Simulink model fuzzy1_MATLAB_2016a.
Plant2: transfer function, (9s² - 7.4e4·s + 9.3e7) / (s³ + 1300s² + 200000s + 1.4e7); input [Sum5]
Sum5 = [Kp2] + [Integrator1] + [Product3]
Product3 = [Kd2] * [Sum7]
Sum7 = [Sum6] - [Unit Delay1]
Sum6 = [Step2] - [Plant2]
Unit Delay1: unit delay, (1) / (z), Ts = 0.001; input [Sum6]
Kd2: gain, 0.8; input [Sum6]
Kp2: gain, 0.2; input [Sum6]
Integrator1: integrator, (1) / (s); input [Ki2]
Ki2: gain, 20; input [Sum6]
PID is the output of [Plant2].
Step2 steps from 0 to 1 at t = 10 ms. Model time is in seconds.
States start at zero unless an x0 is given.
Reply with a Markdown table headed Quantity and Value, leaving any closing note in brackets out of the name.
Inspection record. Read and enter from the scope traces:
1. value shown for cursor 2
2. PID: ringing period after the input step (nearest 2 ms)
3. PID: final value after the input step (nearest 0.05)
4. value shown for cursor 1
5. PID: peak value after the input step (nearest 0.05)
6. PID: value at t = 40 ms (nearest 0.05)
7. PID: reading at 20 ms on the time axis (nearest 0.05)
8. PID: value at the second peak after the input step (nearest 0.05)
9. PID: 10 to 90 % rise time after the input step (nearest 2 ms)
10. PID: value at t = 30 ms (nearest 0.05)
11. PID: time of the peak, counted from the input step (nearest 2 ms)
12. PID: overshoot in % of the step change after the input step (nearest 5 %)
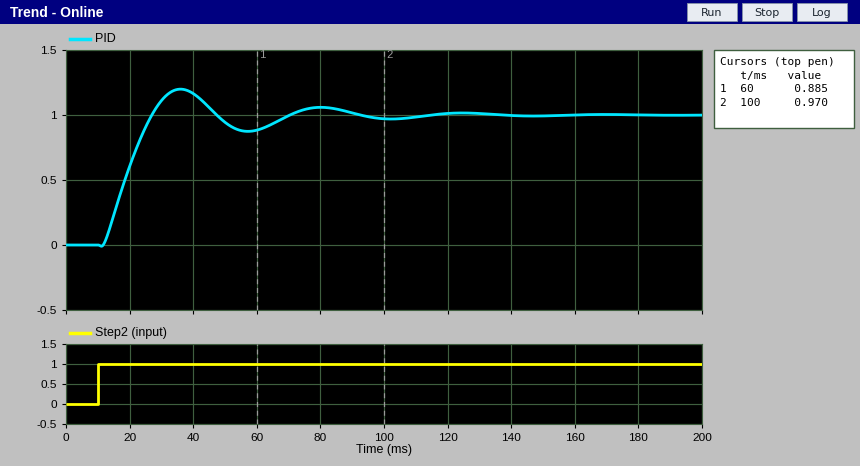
| Quantity | Value |
|---|---|
| value shown for cursor 2 | 0.970 |
| PID: ringing period after the input step | 44 ms |
| PID: final value after the input step | 1.00 |
| value shown for cursor 1 | 0.885 |
| PID: peak value after the input step | 1.20 |
| PID: value at t = 40 ms | 1.15 |
| PID: reading at 20 ms on the time axis | 0.60 |
| PID: value at the second peak after the input step | 1.05 |
| PID: 10 to 90 % rise time after the input step | 12 ms |
| PID: value at t = 30 ms | 1.10 |
| PID: time of the peak, counted from the input step | 26 ms |
| PID: overshoot in % of the step change after the input step | 20 % |
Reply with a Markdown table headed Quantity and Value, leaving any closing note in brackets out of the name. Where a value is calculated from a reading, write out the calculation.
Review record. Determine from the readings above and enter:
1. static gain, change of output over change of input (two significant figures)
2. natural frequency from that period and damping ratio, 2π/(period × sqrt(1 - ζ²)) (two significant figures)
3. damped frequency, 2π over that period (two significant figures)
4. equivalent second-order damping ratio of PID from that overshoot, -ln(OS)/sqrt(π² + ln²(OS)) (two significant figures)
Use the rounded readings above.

| Quantity | Value |
|---|---|
| static gain, change of output over change of input | (1 - 0) / (1 - 0) = 1.0 |
| natural frequency from that period and damping ratio, 2π/(period × sqrt(1 - ζ²)) | 2π / (44 × sqrt(1 - 0.46²)) = 0.16 rad/ms |
| damped frequency, 2π over that period | 2π / 44 = 0.14 rad/ms |
| equivalent second-order damping ratio of PID from that overshoot, -ln(OS)/sqrt(π² + ln²(OS)) | ln(0.2) = -1.609; 1.609 / sqrt(9.870 + 2.590) = 0.46 |
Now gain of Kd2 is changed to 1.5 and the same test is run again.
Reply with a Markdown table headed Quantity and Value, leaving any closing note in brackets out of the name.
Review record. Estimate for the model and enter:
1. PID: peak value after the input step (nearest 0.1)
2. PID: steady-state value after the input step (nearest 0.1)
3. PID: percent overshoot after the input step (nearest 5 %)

| Quantity | Value |
|---|---|
| PID: peak value after the input step | 1.1 |
| PID: steady-state value after the input step | 1.0 |
| PID: percent overshoot after the input step | 10 % |
